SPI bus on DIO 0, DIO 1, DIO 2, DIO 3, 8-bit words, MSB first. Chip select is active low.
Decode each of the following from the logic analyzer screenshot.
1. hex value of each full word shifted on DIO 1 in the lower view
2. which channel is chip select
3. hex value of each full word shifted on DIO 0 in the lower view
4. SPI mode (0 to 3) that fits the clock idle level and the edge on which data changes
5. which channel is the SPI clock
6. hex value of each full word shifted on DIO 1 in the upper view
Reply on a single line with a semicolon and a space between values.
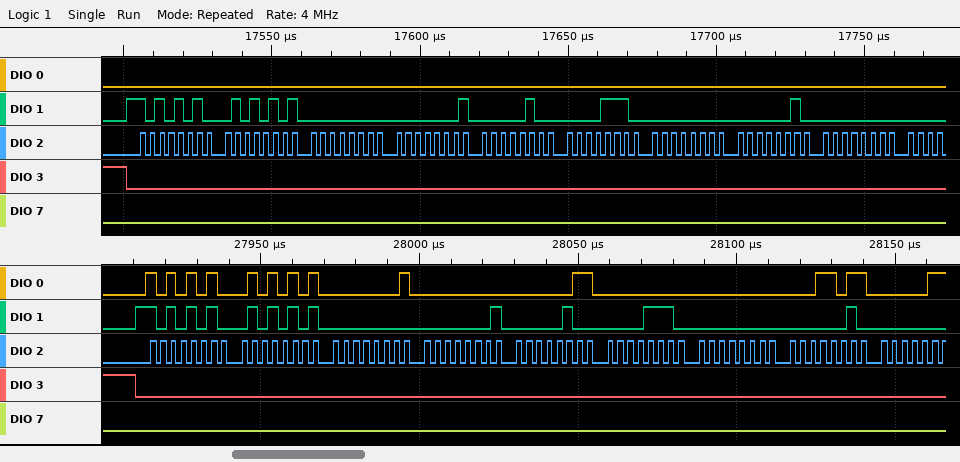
AA, 55, 00, 01, 04, 0E, 00, 02; DIO 3; AA, 55, 01, 00, 03, 00, 00, 1B; 0; DIO 2; AA, 55, 00, 01, 04, 0E, 00, 02, 00
